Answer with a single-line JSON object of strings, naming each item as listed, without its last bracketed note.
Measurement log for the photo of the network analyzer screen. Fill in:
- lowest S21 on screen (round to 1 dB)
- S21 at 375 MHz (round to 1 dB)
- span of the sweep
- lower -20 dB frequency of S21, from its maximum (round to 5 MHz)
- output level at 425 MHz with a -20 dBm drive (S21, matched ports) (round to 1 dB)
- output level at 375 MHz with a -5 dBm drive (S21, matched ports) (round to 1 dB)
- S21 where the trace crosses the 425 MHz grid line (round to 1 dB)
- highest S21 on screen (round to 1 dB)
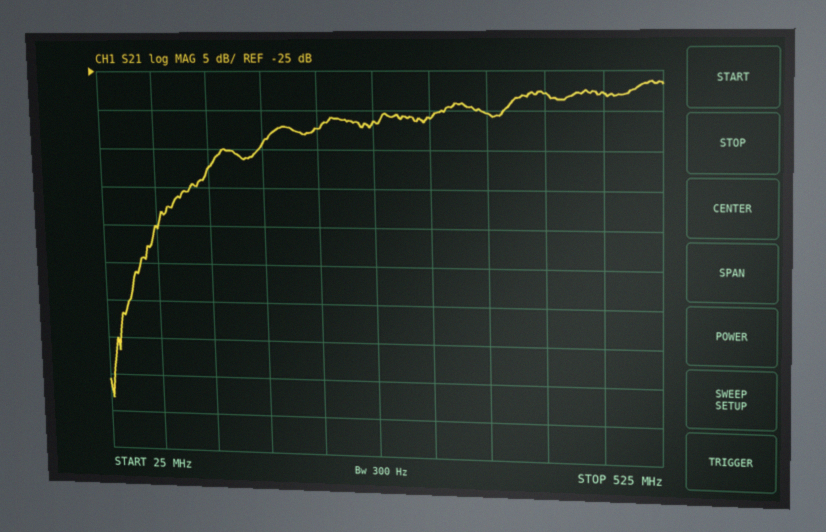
{"lowest S21 on screen": "-68 dB", "S21 at 375 MHz": "-30 dB", "span of the sweep": "500 MHz", "lower -20 dB frequency of S21, from its maximum": "70 MHz", "output level at 425 MHz with a -20 dBm drive (S21, matched ports)": "-48 dBm", "output level at 375 MHz with a -5 dBm drive (S21, matched ports)": "-35 dBm", "S21 where the trace crosses the 425 MHz grid line": "-28 dB", "highest S21 on screen": "-26 dB"}
